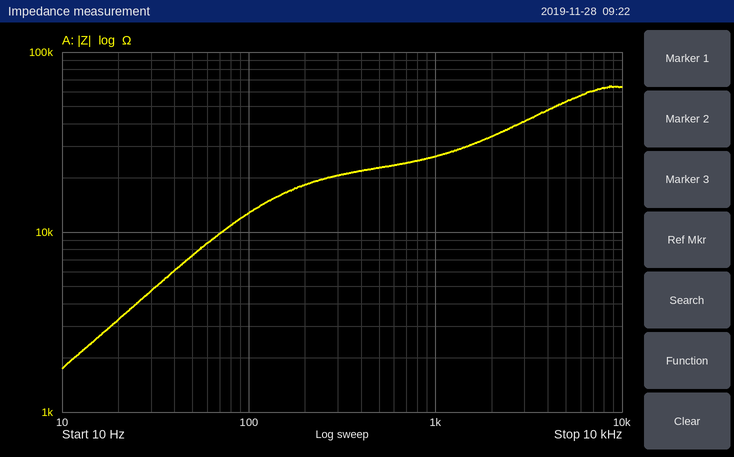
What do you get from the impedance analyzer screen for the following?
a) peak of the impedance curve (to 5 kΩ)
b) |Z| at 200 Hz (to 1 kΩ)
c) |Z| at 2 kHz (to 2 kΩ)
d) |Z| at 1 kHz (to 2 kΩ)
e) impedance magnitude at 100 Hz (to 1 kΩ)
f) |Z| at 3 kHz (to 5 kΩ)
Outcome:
65 kΩ
18 kΩ
34 kΩ
26 kΩ
13 kΩ
40 kΩ
